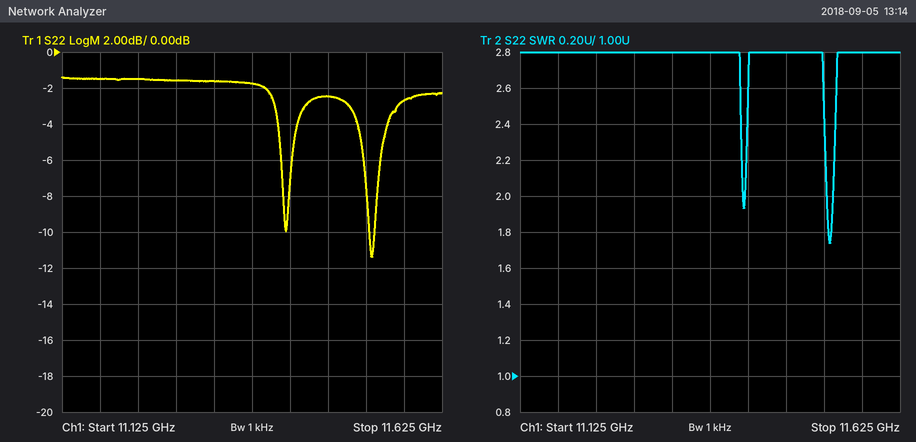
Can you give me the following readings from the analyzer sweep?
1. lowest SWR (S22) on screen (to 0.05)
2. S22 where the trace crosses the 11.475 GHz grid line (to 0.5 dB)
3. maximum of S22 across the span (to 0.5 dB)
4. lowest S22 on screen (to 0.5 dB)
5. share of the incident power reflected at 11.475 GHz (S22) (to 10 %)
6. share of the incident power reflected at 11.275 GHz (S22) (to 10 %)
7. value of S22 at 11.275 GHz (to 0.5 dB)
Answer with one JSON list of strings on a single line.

["1.75", "-2.5 dB", "-1.5 dB", "-11.5 dB", "60 %", "70 %", "-1.5 dB"]
